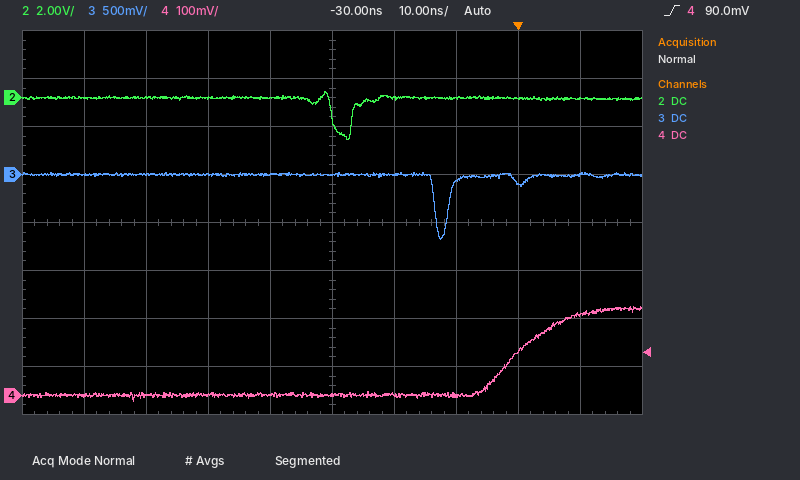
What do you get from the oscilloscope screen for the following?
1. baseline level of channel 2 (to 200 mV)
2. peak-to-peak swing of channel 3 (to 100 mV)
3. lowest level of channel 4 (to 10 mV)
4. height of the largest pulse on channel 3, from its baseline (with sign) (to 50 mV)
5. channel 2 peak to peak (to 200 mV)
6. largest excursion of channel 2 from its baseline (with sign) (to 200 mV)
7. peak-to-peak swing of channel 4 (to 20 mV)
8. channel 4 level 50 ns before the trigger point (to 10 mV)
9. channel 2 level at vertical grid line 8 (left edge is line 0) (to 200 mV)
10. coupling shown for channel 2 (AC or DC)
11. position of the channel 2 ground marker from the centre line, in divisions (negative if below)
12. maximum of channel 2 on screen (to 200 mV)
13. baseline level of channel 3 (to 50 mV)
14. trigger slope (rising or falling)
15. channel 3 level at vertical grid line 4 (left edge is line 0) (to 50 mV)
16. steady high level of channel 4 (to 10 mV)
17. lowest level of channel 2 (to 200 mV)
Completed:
0.0 V
700 mV
-10 mV
-650 mV
2.0 V
-1.8 V
200 mV
0 mV
0.0 V
DC
+2.6 div
200 mV
0 mV
rising
0 mV
180 mV
-1.8 V
